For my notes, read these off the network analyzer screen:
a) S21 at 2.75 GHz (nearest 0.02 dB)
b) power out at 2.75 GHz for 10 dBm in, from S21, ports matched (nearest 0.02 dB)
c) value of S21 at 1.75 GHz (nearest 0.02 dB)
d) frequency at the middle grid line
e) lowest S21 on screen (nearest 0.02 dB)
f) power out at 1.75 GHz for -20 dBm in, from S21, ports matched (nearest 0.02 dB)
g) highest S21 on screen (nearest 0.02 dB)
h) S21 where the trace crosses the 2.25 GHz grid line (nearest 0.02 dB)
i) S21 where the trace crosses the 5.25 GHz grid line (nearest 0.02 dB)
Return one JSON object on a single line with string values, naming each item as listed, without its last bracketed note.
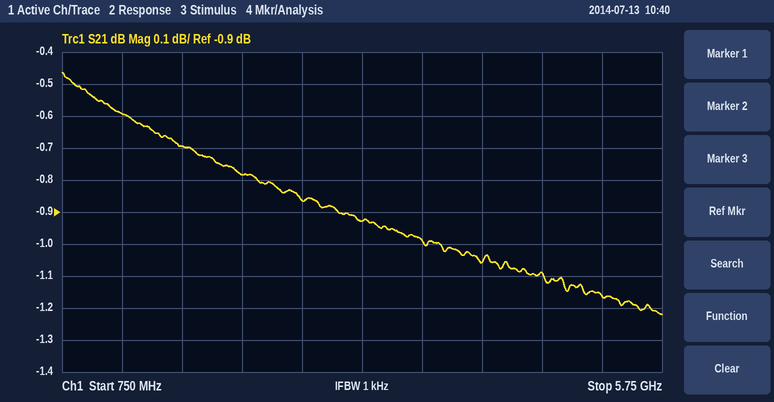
{"S21 at 2.75 GHz": "-0.86 dB", "power out at 2.75 GHz for 10 dBm in, from S21, ports matched": "9.14 dBm", "value of S21 at 1.75 GHz": "-0.70 dB", "frequency at the middle grid line": "3.25 GHz", "lowest S21 on screen": "-1.22 dB", "power out at 1.75 GHz for -20 dBm in, from S21, ports matched": "-20.70 dBm", "highest S21 on screen": "-0.46 dB", "S21 where the trace crosses the 2.25 GHz grid line": "-0.78 dB", "S21 where the trace crosses the 5.25 GHz grid line": "-1.16 dB"}
